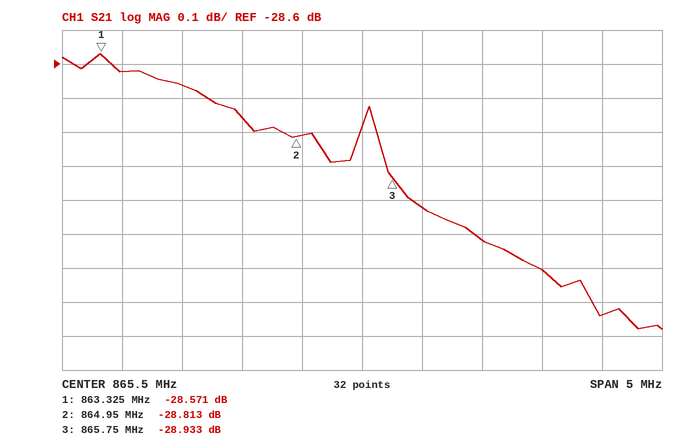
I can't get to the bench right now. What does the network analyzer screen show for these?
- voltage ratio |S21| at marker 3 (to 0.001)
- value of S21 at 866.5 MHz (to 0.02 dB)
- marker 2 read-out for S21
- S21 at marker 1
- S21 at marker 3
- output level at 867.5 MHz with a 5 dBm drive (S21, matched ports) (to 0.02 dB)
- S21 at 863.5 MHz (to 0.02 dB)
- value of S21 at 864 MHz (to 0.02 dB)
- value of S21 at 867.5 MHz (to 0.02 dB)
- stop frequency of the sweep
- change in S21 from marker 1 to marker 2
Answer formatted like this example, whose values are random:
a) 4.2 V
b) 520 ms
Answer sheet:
a) 0.036
b) -29.12 dB
c) -28.813 dB
d) -28.571 dB
e) -28.933 dB
f) -24.34 dBm
g) -28.62 dB
h) -28.66 dB
i) -29.34 dB
j) 868 MHz
k) -0.242 dB
